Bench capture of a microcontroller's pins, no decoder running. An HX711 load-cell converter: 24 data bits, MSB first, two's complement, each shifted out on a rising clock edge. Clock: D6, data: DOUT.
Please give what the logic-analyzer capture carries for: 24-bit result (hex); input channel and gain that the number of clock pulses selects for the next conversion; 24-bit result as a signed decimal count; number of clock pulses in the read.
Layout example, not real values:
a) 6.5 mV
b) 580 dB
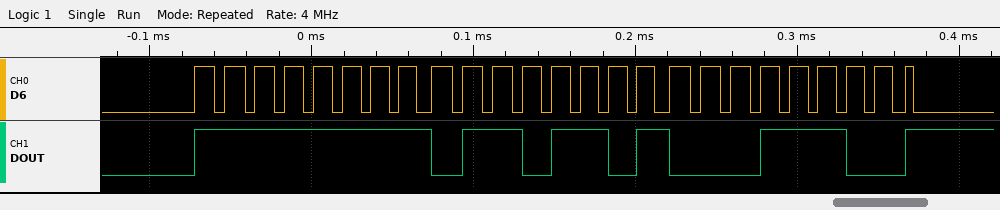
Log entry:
a) 0xFF6D1C
b) channel A, gain 128
c) -37604
d) 25
